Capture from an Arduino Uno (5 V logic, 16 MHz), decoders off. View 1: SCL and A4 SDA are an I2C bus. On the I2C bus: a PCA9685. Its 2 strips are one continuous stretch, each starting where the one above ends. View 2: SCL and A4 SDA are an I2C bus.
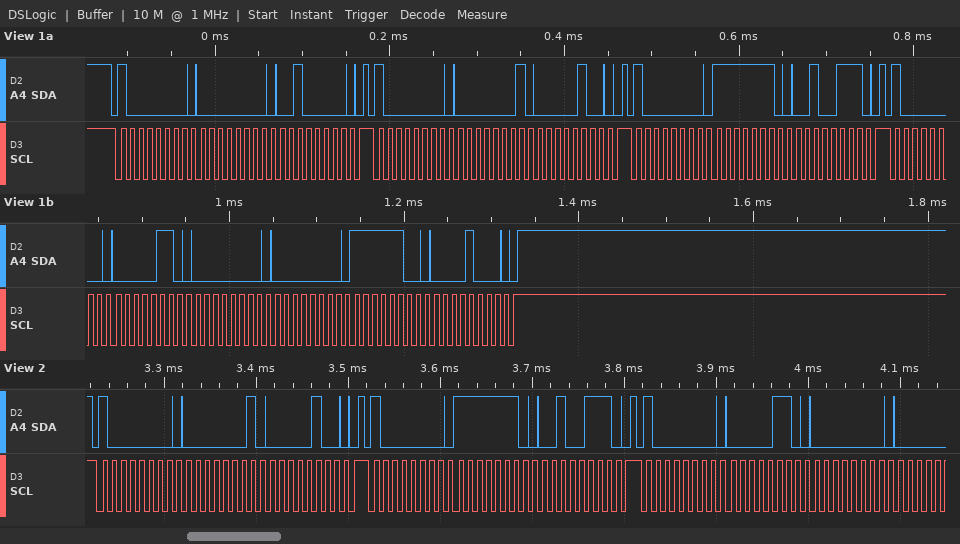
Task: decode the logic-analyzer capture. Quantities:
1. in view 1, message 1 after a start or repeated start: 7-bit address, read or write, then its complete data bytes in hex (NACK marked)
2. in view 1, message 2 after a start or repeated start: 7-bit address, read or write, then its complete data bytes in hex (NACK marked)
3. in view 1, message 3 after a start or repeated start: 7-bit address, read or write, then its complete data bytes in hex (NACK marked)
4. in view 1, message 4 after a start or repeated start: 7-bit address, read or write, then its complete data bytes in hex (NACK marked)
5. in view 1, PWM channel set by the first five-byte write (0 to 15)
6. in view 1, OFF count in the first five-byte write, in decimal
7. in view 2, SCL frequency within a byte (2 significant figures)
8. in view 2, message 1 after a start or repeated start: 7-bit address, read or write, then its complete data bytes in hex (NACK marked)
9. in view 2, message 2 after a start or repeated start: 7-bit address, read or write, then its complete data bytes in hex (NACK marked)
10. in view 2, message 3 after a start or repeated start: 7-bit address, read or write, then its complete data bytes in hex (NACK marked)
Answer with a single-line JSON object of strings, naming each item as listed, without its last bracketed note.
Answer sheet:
{"in view 1, message 1 after a start or repeated start: 7-bit address, read or write, then its complete data bytes in hex": "0x40 write: 00 20", "in view 1, message 2 after a start or repeated start: 7-bit address, read or write, then its complete data bytes in hex": "0x40 write: 01 04", "in view 1, message 3 after a start or repeated start: 7-bit address, read or write, then its complete data bytes in hex": "0x40 write: FE 27", "in view 1, message 4 after a start or repeated start: 7-bit address, read or write, then its complete data bytes in hex": "0x40 write: 06 00 00 FC 08", "in view 1, PWM channel set by the first five-byte write": "0", "in view 1, OFF count in the first five-byte write, in decimal": "2300", "in view 2, SCL frequency within a byte": "100 kHz", "in view 2, message 1 after a start or repeated start: 7-bit address, read or write, then its complete data bytes in hex": "0x40 write: 01 04", "in view 2, message 2 after a start or repeated start: 7-bit address, read or write, then its complete data bytes in hex": "0x40 write: FE 27", "in view 2, message 3 after a start or repeated start: 7-bit address, read or write, then its complete data bytes in hex": "0x40 write: 06 00"}
